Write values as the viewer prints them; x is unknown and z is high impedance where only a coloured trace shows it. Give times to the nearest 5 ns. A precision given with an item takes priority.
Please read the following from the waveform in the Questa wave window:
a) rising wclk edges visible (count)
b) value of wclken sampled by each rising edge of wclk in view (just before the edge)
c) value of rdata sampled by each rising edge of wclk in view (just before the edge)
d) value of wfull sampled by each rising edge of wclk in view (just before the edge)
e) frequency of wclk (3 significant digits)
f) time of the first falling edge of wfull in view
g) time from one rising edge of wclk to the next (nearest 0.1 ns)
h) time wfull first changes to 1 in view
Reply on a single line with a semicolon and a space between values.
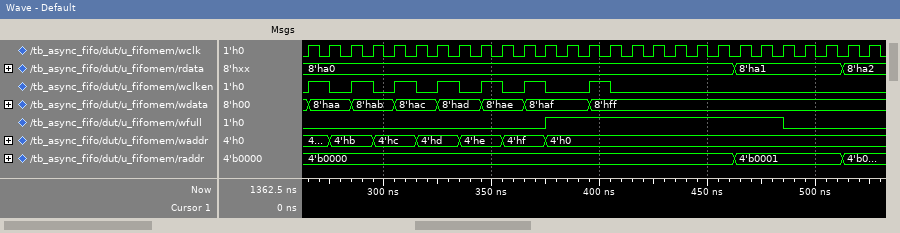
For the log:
27; 0 1 0 1 0 1 0 1 0 1 0 1 0 0 1 0 0 0 0 0 0 0 0 0 0 0 0; 8'ha0, 8'ha0, 8'ha0, 8'ha0, 8'ha0, 8'ha0, 8'ha0, 8'ha0, 8'ha0, 8'ha0, 8'ha0, 8'ha0, 8'ha0, 8'ha0, 8'ha0, 8'ha0, 8'ha0, 8'ha0, 8'ha0, 8'ha0, 8'ha1, 8'ha1, 8'ha1, 8'ha1, 8'ha1, 8'ha2, 8'ha2; 0 0 0 0 0 0 0 0 0 0 0 0 1 1 1 1 1 1 1 1 1 1 1 0 0 0 0; 100 MHz; 485 ns; 10 ns; 375 ns
